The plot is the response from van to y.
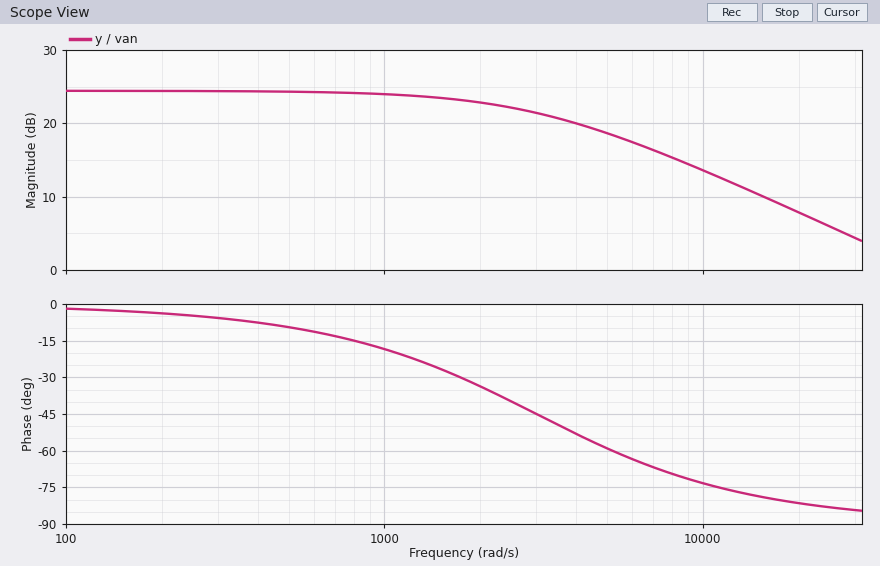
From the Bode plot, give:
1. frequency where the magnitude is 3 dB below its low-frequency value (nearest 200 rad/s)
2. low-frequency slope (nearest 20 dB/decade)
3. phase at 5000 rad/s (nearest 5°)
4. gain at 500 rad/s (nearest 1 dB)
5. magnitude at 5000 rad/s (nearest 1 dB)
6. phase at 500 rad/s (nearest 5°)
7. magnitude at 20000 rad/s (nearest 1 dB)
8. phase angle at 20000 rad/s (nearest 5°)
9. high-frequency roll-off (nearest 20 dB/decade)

3000 rad/s
0 dB/decade
-60°
24 dB
19 dB
-10°
8 dB
-80°
-20 dB/decade
